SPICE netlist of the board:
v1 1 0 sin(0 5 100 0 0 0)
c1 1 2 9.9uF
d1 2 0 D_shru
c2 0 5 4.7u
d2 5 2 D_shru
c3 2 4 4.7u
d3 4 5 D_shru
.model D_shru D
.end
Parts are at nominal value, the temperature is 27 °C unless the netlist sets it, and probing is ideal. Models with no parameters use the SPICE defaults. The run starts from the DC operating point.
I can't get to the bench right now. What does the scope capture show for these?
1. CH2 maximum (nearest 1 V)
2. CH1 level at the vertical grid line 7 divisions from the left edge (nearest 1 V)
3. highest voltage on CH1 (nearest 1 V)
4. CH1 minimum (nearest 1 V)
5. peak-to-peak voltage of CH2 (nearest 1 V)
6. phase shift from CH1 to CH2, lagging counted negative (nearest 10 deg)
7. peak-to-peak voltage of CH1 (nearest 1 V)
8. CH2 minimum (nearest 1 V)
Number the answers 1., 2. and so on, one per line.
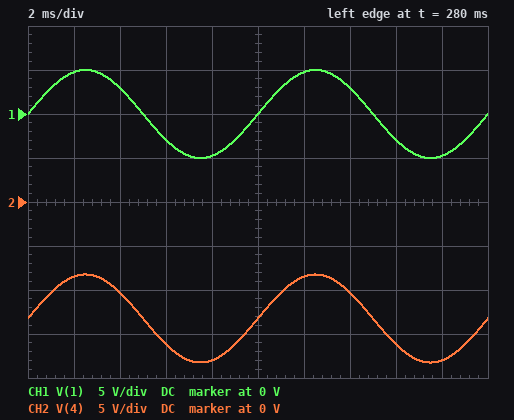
1. -8 V
2. 3 V
3. 5 V
4. -5 V
5. 10 V
6. 0 deg
7. 10 V
8. -18 V
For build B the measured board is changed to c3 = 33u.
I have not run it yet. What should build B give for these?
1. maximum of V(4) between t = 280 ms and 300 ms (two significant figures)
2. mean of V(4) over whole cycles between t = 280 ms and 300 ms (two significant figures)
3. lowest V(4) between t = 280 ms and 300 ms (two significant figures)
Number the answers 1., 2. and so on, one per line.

1. -7.4 V
2. -12 V
3. -17 V
